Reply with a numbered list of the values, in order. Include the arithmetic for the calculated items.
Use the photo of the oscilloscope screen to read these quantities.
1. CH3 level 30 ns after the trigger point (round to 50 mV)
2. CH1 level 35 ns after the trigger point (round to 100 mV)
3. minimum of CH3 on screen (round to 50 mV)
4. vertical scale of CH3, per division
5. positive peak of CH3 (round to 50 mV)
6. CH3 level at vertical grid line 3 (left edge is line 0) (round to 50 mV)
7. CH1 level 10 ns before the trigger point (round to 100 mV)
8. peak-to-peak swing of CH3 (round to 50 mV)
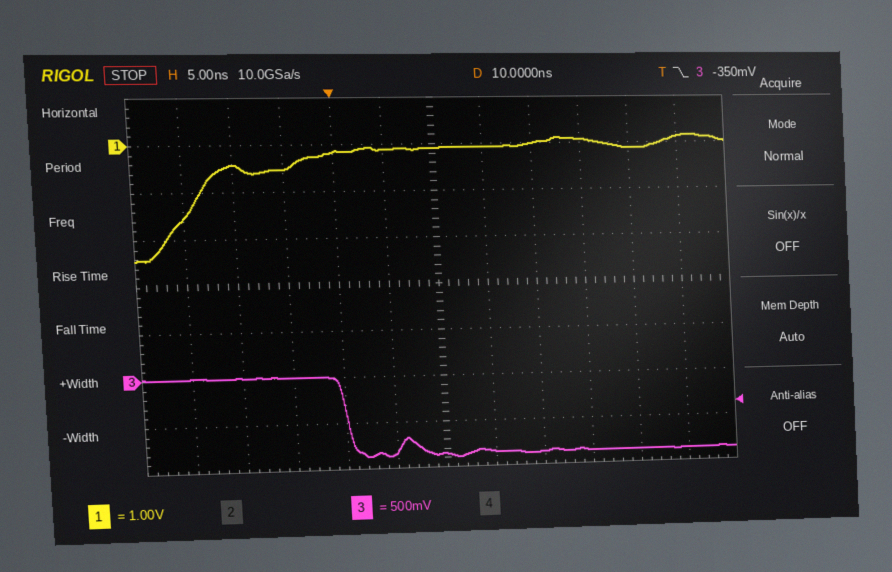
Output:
1. -850 mV
2. 100 mV
3. -900 mV
4. 500 mV
5. 0 mV
6. 0 mV
7. -400 mV
8. 0 mV − (-900 mV) = 900 mV
